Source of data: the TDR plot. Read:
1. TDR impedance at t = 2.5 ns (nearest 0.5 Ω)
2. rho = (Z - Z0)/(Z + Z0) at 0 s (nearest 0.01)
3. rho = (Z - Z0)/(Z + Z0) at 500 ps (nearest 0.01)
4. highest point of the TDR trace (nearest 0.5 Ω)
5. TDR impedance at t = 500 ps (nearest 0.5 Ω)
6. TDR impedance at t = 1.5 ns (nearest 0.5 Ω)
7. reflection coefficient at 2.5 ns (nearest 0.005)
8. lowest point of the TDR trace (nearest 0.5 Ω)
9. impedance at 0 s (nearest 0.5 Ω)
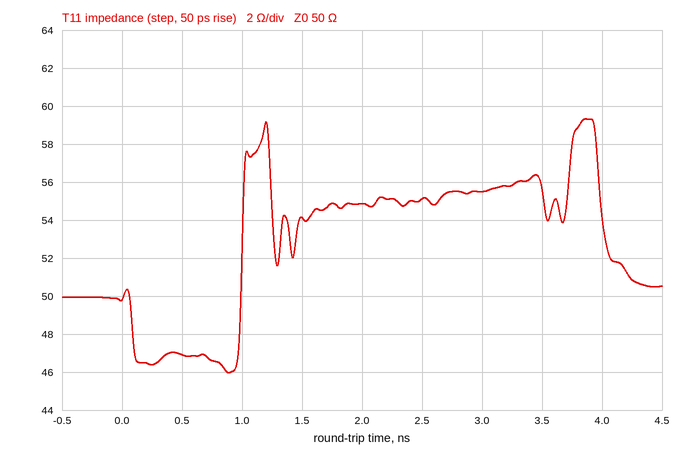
55.0 Ω
0.00
-0.03
59.5 Ω
47.0 Ω
54.0 Ω
+0.050
46.0 Ω
50.0 Ω
